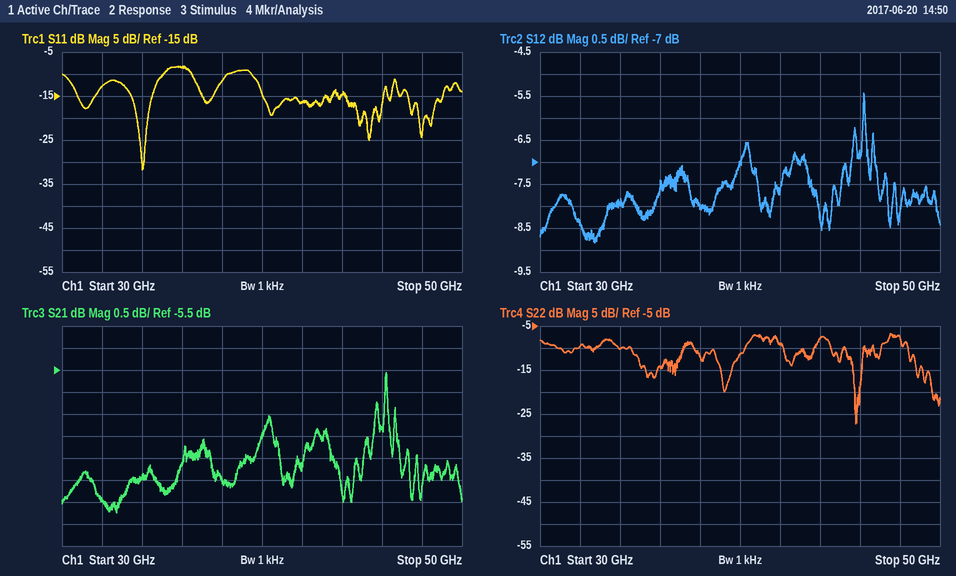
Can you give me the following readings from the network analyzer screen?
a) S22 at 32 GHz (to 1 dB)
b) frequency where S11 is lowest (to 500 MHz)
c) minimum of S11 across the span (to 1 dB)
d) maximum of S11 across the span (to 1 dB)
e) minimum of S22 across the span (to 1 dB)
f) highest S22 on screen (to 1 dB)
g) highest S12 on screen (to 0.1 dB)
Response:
-10 dB
34.0 GHz
-32 dB
-8 dB
-27 dB
-7 dB
-5.4 dB
